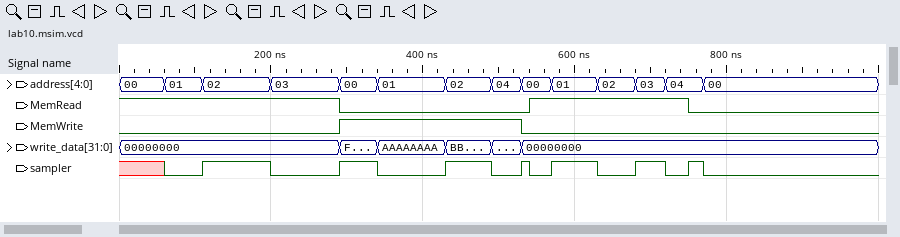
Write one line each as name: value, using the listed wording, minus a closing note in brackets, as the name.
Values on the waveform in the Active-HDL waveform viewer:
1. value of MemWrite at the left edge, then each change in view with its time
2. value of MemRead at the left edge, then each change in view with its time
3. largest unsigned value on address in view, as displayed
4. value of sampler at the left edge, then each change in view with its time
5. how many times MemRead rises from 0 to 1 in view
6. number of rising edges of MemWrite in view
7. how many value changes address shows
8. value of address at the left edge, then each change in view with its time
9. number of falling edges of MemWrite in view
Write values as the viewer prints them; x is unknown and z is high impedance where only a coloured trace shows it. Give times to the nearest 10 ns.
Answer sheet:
value of MemWrite at the left edge, then each change in view with its time: 0, 1 at 290 ns, 0 at 530 ns
value of MemRead at the left edge, then each change in view with its time: 1, 0 at 290 ns, 1 at 540 ns, 0 at 750 ns
largest unsigned value on address in view, as displayed: 04
value of sampler at the left edge, then each change in view with its time: x, 0 at 60 ns, 1 at 110 ns, 0 at 200 ns, 1 at 290 ns, 0 at 340 ns, 1 at 430 ns, 0 at 490 ns, 1 at 530 ns, 0 at 540 ns, 1 at 570 ns, 0 at 630 ns, 1 at 680 ns, 0 at 720 ns, 1 at 750 ns, 0 at 770 ns
how many times MemRead rises from 0 to 1 in view: 1
number of rising edges of MemWrite in view: 1
how many value changes address shows: 13
value of address at the left edge, then each change in view with its time: 00, 01 at 60 ns, 02 at 110 ns, 03 at 200 ns, 00 at 290 ns, 01 at 340 ns, 02 at 430 ns, 04 at 490 ns, 00 at 530 ns, 01 at 570 ns, 02 at 630 ns, 03 at 680 ns, 04 at 720 ns, 00 at 770 ns
number of falling edges of MemWrite in view: 1
